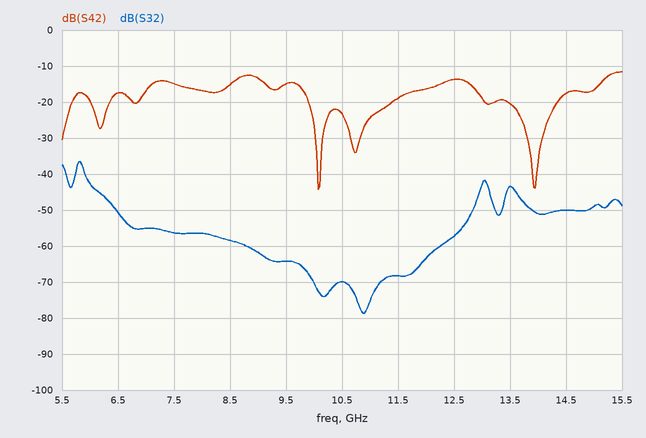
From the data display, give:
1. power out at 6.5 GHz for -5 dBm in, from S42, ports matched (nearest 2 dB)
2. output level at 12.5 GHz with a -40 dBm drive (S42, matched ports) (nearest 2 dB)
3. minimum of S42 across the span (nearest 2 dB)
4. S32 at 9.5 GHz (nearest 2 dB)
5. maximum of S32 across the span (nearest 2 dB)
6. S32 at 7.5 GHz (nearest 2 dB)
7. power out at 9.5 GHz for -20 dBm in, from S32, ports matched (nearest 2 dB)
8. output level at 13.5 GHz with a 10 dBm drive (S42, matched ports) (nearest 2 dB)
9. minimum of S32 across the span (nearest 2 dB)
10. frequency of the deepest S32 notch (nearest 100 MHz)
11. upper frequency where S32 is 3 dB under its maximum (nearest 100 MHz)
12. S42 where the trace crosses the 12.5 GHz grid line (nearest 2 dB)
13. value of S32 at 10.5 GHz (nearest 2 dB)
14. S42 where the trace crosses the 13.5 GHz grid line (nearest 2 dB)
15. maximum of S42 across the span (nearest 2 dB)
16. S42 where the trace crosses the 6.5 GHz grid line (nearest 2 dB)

-22 dBm
-54 dBm
-44 dB
-64 dB
-36 dB
-56 dB
-84 dBm
-10 dBm
-78 dB
10.9 GHz
5.9 GHz
-14 dB
-70 dB
-20 dB
-12 dB
-18 dB
